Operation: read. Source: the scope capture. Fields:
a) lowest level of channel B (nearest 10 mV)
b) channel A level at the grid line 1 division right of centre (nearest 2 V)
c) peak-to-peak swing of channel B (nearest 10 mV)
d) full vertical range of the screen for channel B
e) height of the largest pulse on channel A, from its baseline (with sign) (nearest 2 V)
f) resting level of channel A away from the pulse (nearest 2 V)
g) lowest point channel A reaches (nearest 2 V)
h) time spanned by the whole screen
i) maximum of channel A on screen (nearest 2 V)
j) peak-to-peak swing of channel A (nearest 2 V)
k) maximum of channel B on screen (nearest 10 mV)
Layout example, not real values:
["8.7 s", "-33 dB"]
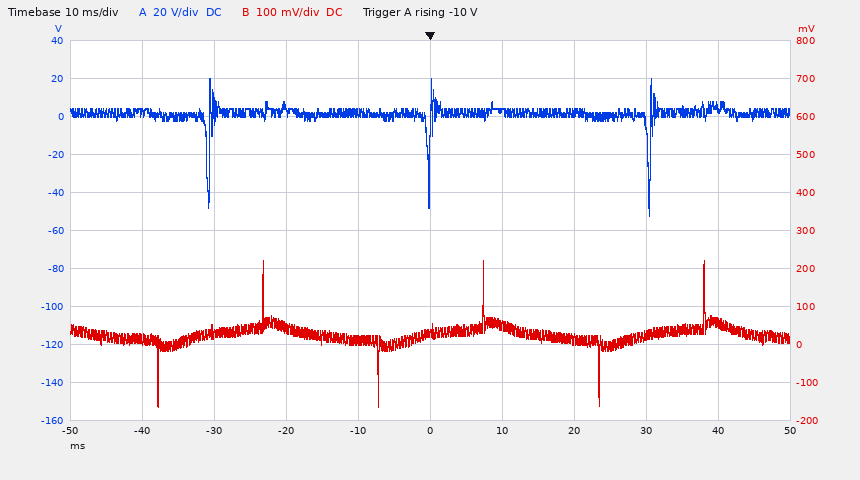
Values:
["-160 mV", "2 V", "380 mV", "1 V", "-54 V", "2 V", "-52 V", "100 ms", "20 V", "72 V", "220 mV"]
